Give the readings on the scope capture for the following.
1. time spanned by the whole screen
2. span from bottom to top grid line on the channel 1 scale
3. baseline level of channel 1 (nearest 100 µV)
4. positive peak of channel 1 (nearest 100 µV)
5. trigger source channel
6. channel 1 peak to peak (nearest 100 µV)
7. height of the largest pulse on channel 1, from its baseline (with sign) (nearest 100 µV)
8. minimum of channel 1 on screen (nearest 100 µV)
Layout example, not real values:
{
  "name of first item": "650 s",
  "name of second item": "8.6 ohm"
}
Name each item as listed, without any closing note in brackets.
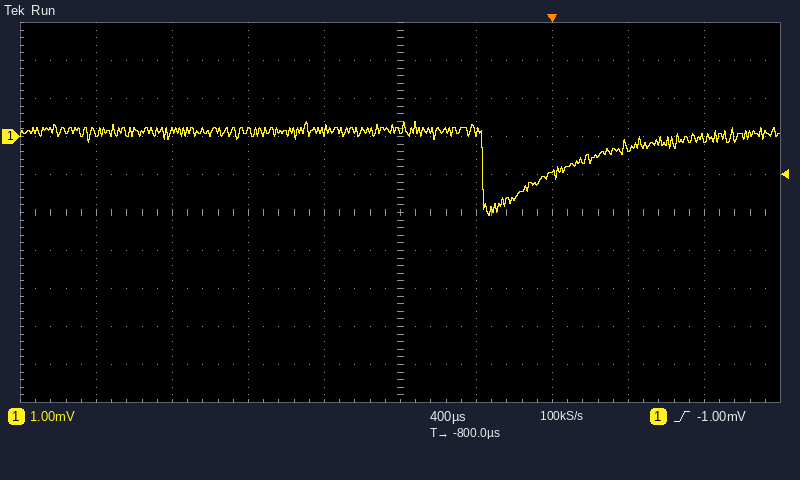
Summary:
{
  "time spanned by the whole screen": "4 ms",
  "span from bottom to top grid line on the channel 1 scale": "10 mV",
  "baseline level of channel 1": "100 µV",
  "positive peak of channel 1": "400 µV",
  "trigger source channel": "channel 1",
  "channel 1 peak to peak": "2.5 mV",
  "height of the largest pulse on channel 1, from its baseline (with sign)": "-2.2 mV",
  "minimum of channel 1 on screen": "-2.1 mV"
}
